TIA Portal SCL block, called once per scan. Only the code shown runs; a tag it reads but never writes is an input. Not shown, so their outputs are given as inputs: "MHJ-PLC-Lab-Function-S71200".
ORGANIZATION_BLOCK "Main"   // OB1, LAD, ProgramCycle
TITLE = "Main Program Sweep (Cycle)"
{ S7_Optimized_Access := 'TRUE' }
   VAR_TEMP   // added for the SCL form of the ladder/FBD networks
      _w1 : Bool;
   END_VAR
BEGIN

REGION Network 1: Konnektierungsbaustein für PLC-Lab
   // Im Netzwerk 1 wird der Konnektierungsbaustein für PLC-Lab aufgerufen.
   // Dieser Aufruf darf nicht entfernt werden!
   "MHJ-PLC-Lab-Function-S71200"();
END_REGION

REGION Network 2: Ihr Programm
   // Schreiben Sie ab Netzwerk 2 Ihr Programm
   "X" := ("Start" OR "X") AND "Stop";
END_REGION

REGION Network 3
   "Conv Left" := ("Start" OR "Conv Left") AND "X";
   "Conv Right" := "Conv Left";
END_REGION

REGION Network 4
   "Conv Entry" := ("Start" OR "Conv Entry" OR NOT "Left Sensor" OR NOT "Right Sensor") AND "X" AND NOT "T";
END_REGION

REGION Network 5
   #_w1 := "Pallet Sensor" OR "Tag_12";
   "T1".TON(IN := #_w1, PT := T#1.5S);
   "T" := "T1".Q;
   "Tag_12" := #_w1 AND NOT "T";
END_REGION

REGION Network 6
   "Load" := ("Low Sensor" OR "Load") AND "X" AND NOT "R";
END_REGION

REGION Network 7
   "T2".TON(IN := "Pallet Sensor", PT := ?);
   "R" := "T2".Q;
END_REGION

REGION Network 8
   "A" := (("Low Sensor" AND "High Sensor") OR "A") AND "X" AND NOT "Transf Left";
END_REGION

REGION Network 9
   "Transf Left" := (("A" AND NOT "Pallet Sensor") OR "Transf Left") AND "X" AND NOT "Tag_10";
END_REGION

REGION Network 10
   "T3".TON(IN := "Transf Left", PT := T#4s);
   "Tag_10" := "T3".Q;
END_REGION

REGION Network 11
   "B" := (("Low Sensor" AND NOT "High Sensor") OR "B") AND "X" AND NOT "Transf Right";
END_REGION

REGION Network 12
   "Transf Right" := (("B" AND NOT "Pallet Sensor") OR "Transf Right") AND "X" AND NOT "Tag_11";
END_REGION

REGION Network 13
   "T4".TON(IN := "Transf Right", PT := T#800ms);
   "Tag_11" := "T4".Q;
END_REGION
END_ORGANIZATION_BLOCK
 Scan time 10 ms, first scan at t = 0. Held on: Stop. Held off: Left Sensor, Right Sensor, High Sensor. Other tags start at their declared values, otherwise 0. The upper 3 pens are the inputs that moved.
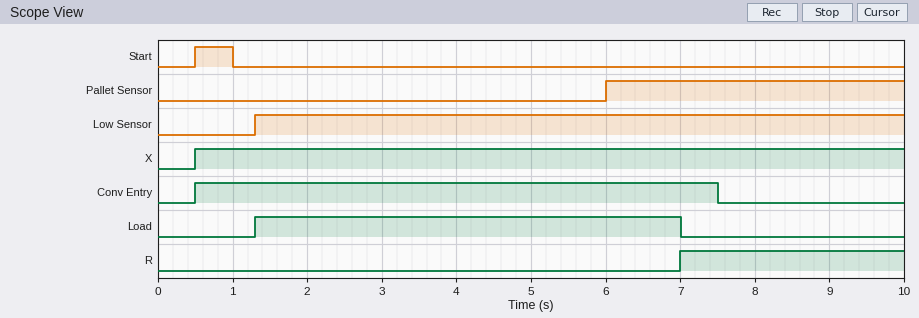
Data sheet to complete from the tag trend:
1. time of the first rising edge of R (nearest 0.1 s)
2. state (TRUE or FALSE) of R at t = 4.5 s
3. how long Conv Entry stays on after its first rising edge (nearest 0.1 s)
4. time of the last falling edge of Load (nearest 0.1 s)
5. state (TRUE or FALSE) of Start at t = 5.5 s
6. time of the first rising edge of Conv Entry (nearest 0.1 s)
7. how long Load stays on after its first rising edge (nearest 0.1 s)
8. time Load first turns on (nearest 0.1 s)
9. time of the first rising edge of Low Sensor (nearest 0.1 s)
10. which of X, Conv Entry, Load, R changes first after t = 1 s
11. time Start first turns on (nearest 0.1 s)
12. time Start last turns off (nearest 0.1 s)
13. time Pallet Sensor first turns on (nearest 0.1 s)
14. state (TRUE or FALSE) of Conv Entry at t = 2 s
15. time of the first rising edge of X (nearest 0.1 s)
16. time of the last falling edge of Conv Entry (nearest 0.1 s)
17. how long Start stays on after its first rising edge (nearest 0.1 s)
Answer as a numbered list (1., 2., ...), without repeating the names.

1. 7.0 s
2. FALSE
3. 7.0 s
4. 7.0 s
5. FALSE
6. 0.5 s
7. 5.7 s
8. 1.3 s
9. 1.3 s
10. Load
11. 0.5 s
12. 1.0 s
13. 6.0 s
14. TRUE
15. 0.5 s
16. 7.5 s
17. 0.5 s
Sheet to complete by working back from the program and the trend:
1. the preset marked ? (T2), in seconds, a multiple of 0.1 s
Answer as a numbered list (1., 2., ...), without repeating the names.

1. 1.0 s
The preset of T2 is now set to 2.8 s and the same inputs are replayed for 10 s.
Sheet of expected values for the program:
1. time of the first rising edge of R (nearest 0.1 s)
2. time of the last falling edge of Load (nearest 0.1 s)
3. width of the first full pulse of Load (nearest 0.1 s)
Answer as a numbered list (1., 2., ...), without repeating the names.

1. 8.8 s
2. 8.8 s
3. 7.5 s
